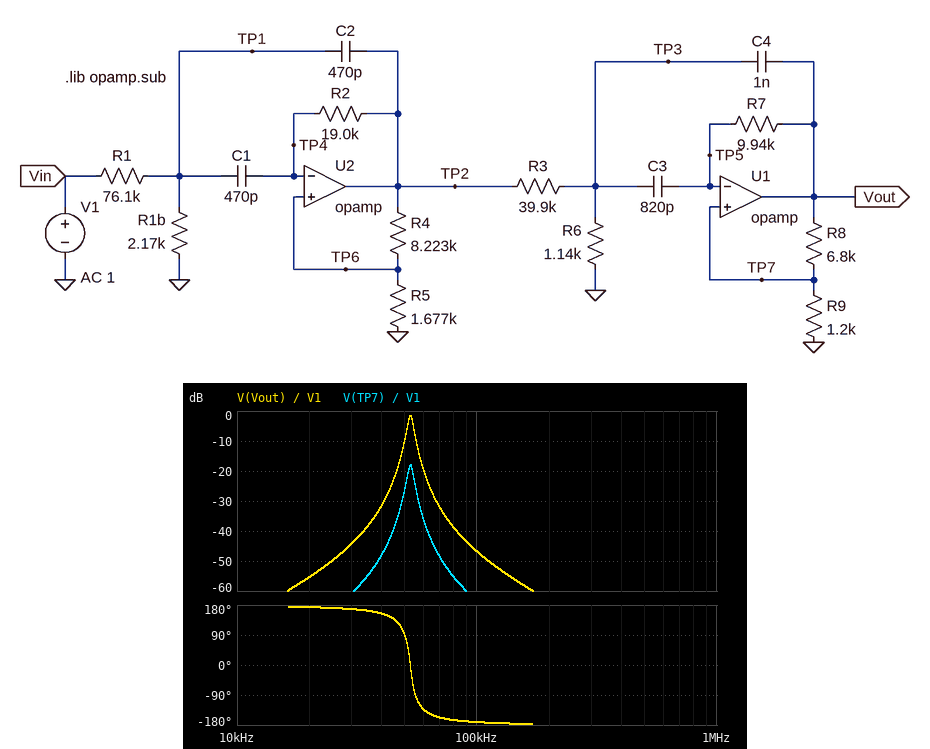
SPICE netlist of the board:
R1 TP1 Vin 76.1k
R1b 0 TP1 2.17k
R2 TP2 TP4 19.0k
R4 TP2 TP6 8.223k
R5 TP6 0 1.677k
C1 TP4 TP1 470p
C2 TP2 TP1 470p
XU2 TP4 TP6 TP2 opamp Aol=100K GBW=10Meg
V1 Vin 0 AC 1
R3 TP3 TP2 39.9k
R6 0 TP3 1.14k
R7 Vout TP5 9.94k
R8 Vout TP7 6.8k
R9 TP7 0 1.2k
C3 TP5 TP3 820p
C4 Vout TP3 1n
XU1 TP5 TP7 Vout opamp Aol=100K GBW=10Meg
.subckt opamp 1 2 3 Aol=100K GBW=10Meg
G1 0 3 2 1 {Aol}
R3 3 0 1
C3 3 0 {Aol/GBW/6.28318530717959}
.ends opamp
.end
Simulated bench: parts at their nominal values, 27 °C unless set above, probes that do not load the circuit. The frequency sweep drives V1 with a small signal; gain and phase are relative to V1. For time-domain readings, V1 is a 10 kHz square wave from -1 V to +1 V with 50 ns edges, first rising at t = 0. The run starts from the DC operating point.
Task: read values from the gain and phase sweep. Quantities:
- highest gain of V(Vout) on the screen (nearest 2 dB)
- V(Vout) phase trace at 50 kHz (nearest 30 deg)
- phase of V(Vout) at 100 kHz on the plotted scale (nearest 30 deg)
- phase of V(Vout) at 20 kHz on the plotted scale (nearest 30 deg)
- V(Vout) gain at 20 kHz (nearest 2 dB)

-2 dB
90 deg
-180 deg
180 deg
-56 dB
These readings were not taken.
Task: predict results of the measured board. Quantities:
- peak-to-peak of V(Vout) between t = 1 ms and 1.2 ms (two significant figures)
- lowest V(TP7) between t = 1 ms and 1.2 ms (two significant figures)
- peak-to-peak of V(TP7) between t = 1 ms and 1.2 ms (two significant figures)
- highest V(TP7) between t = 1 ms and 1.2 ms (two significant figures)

170 mV
-13 mV
26 mV
13 mV
